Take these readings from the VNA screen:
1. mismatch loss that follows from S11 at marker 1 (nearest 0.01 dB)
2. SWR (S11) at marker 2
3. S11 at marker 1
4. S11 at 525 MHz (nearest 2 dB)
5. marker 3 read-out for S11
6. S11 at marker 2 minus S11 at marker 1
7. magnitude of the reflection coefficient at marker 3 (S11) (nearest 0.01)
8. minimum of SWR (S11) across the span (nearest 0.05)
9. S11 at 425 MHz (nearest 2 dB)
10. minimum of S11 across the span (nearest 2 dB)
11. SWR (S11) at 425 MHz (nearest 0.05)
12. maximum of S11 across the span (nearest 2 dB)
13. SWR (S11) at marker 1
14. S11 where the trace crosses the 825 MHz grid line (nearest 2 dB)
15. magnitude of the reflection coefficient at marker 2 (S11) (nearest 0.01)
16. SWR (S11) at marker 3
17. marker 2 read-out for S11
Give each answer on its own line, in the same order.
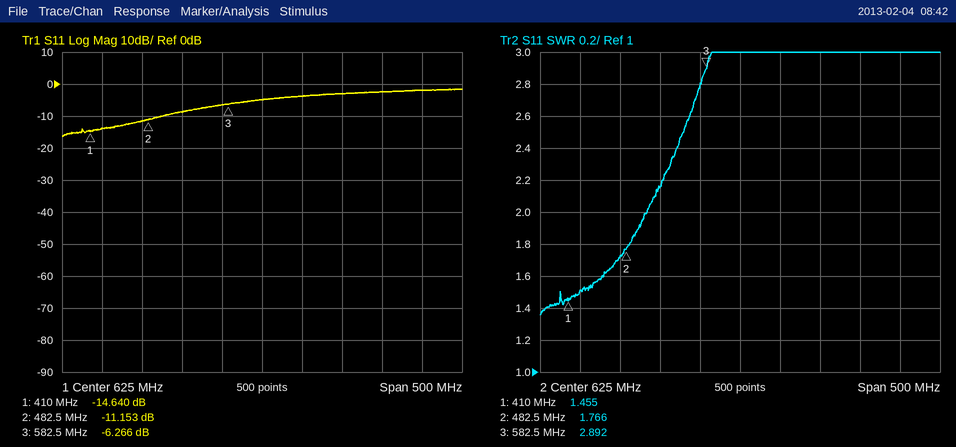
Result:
0.15 dB
1.766
-14.640 dB
-8 dB
-6.266 dB
3.487 dB
0.49
1.35
-14 dB
-16 dB
1.50
-2 dB
1.455
-2 dB
0.28
2.892
-11.153 dB
